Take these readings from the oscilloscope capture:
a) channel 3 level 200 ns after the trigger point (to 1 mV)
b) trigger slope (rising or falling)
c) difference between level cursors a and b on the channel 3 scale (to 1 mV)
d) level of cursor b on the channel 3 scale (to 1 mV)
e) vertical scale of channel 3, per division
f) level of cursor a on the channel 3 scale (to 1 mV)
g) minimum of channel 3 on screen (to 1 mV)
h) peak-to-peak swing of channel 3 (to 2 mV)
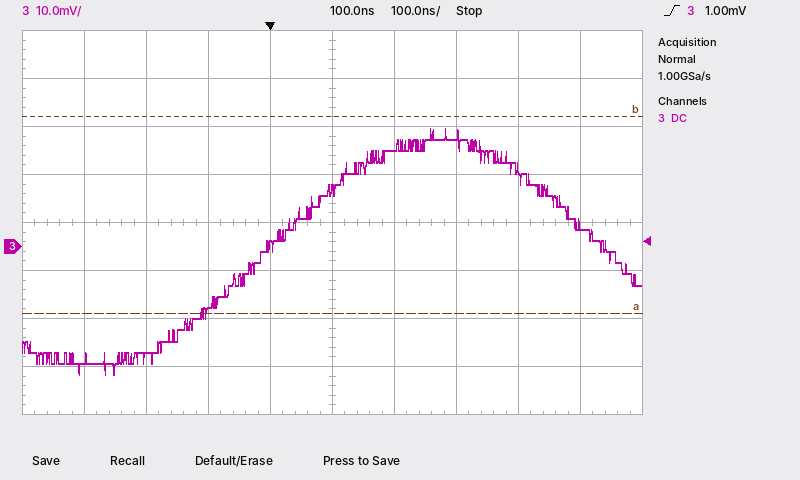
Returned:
21 mV
rising
41 mV
27 mV
10 mV
-14 mV
-27 mV
52 mV
